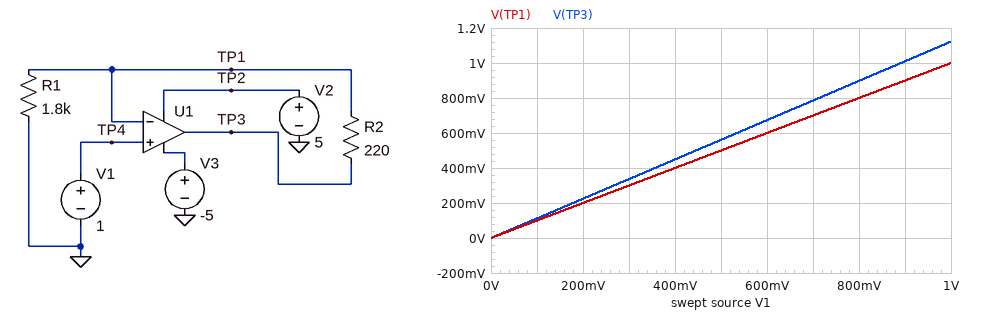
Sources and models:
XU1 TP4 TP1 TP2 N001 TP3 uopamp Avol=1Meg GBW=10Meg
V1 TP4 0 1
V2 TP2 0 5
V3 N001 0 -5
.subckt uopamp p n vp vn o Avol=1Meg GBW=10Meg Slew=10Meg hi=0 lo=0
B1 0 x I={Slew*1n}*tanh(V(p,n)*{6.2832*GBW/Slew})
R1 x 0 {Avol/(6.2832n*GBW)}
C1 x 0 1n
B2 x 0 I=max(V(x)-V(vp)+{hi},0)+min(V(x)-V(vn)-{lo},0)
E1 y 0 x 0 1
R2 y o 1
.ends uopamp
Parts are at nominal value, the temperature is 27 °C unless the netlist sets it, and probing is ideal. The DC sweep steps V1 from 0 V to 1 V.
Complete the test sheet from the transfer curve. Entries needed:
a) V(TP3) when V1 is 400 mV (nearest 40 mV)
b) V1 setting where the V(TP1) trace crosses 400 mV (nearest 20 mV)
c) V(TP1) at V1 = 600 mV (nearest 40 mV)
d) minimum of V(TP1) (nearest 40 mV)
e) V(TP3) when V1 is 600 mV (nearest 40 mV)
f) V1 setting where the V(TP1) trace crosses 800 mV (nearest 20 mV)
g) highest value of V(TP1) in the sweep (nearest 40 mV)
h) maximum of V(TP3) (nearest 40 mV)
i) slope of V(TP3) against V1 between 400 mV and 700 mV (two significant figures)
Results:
440 mV
400 mV
600 mV
0 V
680 mV
800 mV
1.00 V
1.12 V
1.1 V/V
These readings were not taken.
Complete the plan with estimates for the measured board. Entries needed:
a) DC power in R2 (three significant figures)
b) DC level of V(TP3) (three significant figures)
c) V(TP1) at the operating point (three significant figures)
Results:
67.9 µW
1.12 V
1.00 V
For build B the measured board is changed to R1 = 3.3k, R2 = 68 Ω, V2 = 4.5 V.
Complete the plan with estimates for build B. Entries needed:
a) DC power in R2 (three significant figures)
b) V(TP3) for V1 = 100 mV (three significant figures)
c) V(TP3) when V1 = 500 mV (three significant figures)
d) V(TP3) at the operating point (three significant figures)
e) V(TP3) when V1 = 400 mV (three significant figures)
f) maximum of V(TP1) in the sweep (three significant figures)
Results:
6.24 µW
102 mV
510 mV
1.02 V
408 mV
1.00 V
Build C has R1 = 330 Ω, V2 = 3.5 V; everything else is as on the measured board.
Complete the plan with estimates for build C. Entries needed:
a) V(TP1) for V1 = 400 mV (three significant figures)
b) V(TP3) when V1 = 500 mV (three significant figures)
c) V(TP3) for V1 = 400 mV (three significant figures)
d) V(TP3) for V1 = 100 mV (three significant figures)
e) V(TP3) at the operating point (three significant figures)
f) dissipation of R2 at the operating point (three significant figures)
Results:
400 mV
833 mV
667 mV
167 mV
1.67 V
2.02 mW
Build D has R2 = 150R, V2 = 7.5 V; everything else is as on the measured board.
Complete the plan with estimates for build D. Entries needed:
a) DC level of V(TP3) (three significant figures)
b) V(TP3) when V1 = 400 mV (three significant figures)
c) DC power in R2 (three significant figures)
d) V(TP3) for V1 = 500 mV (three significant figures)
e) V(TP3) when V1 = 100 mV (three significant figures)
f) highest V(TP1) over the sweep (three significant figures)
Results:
1.08 V
433 mV
46.3 µW
542 mV
108 mV
1.00 V
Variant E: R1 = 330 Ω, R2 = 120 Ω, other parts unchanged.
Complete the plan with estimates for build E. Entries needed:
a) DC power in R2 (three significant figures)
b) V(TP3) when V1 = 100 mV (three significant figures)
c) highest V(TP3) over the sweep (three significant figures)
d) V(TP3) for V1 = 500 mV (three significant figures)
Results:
1.10 mW
136 mV
1.36 V
682 mV
